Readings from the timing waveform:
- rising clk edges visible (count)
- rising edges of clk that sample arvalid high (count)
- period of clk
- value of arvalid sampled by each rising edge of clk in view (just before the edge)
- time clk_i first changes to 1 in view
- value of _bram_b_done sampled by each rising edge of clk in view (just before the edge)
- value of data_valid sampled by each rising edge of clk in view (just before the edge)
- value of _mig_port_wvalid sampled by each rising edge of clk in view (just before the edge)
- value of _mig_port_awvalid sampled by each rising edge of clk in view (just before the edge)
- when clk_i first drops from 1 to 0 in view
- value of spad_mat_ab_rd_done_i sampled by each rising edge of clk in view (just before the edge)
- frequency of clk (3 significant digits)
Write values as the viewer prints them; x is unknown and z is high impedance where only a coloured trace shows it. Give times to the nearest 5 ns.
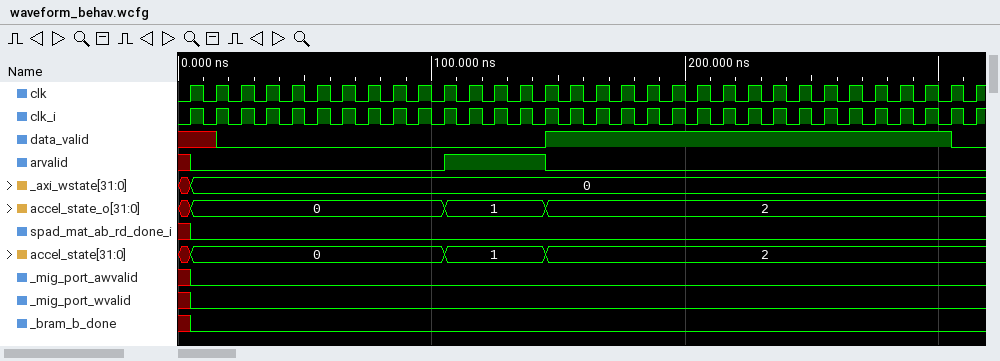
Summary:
32
4
10 ns
x 0 0 0 0 0 0 0 0 0 0 1 1 1 1 0 0 0 0 0 0 0 0 0 0 0 0 0 0 0 0 0
5 ns
x 0 0 0 0 0 0 0 0 0 0 0 0 0 0 0 0 0 0 0 0 0 0 0 0 0 0 0 0 0 0 0
x x 0 0 0 0 0 0 0 0 0 0 0 0 0 1 1 1 1 1 1 1 1 1 1 1 1 1 1 1 1 0
x 0 0 0 0 0 0 0 0 0 0 0 0 0 0 0 0 0 0 0 0 0 0 0 0 0 0 0 0 0 0 0
x 0 0 0 0 0 0 0 0 0 0 0 0 0 0 0 0 0 0 0 0 0 0 0 0 0 0 0 0 0 0 0
10 ns
x 0 0 0 0 0 0 0 0 0 0 0 0 0 0 0 0 0 0 0 0 0 0 0 0 0 0 0 0 0 0 0
100 MHz
